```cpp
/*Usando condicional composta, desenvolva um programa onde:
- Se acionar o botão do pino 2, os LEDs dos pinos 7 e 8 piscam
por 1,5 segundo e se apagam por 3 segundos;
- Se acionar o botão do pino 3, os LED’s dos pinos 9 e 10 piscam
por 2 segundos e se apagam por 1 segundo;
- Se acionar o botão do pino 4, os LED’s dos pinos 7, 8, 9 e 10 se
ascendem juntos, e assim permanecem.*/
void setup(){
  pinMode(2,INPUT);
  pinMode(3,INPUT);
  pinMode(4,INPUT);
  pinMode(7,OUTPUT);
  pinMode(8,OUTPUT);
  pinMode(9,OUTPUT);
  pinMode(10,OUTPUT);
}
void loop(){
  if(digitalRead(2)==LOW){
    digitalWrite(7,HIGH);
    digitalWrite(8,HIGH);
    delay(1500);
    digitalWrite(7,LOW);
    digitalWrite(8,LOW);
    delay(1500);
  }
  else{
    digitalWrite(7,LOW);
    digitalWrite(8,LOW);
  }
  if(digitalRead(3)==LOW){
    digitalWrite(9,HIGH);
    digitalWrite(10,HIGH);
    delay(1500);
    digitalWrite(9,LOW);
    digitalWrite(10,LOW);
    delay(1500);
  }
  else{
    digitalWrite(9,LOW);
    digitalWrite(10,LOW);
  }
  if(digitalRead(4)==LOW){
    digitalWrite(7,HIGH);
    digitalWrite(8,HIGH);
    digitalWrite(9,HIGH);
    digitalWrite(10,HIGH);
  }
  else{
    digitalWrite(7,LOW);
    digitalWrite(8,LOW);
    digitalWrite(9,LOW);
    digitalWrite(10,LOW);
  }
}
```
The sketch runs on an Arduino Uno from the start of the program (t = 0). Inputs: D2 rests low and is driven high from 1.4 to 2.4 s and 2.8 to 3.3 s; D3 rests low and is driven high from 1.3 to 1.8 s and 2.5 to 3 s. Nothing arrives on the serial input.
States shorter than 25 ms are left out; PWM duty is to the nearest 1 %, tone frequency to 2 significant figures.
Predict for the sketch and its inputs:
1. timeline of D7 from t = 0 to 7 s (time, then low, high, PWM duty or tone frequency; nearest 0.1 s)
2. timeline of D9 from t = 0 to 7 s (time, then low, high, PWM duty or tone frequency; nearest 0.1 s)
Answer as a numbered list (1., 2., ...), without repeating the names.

1. 0 s high; 1.5 s low; 6 s high
2. 0 s low; 3 s high; 4.5 s low; 6 s high
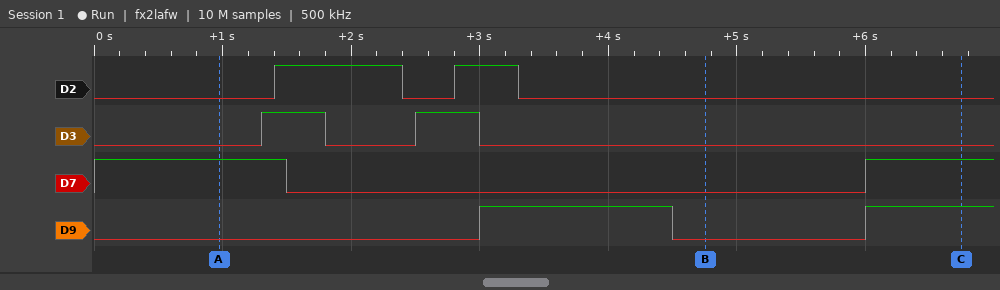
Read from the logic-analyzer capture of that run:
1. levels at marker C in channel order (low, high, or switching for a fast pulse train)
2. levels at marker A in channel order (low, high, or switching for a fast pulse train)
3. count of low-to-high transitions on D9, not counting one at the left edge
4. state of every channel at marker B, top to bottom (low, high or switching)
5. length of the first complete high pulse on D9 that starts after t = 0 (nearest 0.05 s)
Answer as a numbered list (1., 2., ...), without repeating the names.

1. D2 low, D3 low, D7 high, D9 high
2. D2 low, D3 low, D7 high, D9 low
3. 2
4. D2 low, D3 low, D7 low, D9 low
5. 1.50 s
